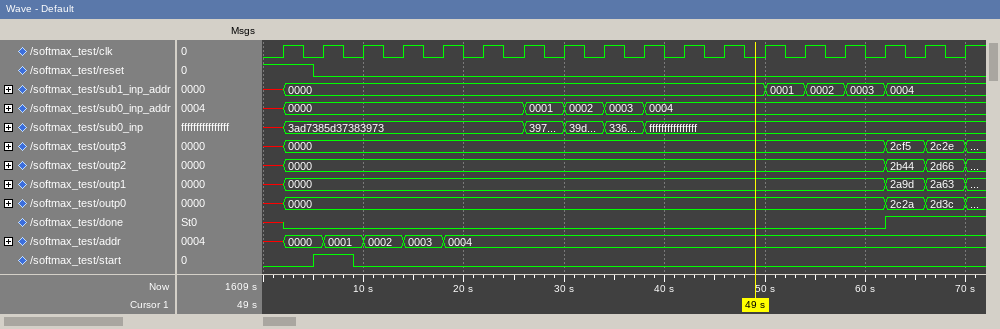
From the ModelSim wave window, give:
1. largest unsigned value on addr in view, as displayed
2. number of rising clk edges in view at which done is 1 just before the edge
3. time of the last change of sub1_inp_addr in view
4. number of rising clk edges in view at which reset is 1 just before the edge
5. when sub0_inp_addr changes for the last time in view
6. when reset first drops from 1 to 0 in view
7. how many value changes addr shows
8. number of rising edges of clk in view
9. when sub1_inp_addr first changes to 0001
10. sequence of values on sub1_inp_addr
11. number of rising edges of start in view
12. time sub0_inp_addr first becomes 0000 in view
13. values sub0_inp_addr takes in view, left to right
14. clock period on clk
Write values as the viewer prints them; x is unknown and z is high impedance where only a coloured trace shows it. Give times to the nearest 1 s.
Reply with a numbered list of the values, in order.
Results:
1. 0004
2. 2
3. 62 s
4. 1
5. 38 s
6. 5 s
7. 5
8. 18
9. 50 s
10. x, 0000, 0001, 0002, 0003, 0004
11. 1
12. 2 s
13. x, 0000, 0001, 0002, 0003, 0004
14. 4 s
